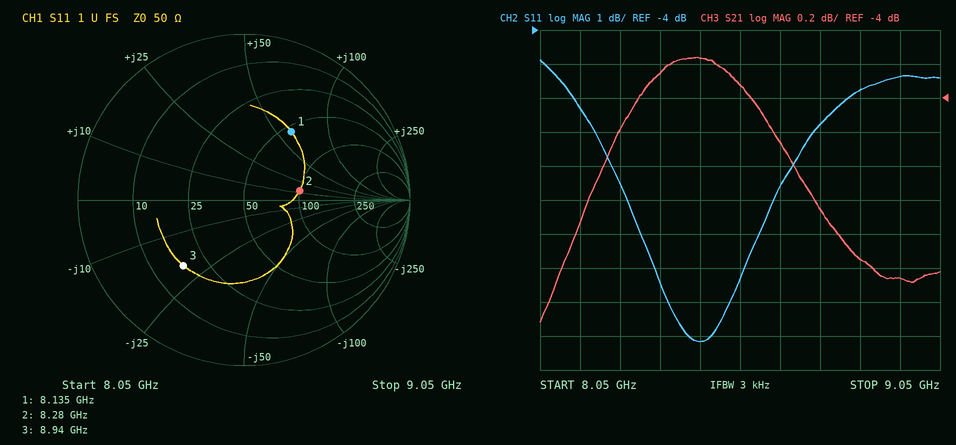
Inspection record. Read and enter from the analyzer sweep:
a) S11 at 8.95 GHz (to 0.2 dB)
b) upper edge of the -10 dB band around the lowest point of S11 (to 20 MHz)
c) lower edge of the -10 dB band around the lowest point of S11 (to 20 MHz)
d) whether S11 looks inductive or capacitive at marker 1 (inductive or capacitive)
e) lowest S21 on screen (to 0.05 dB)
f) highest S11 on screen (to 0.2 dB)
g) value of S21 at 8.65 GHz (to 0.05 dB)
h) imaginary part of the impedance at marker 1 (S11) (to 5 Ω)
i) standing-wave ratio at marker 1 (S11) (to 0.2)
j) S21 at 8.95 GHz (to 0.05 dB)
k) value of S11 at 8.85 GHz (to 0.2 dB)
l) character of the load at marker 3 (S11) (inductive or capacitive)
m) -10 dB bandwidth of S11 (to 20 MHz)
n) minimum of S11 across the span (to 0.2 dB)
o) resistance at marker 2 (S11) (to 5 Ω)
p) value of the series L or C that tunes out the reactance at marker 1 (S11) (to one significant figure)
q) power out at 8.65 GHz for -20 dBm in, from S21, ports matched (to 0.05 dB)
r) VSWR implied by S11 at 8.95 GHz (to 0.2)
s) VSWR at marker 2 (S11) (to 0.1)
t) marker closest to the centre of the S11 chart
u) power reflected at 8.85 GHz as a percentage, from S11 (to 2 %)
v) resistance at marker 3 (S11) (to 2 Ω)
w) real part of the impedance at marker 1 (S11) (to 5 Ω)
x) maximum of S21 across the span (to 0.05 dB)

-5.4 dB
8.60 GHz
8.30 GHz
inductive
-5.30 dB
-4.8 dB
-4.25 dB
+60 Ω
3.0
-5.05 dB
-5.8 dB
capacitive
300 MHz
-13.2 dB
100 Ω
300 fF
-24.25 dBm
3.4
2.0
marker 2
26 %
18 Ω
55 Ω
-3.75 dB
